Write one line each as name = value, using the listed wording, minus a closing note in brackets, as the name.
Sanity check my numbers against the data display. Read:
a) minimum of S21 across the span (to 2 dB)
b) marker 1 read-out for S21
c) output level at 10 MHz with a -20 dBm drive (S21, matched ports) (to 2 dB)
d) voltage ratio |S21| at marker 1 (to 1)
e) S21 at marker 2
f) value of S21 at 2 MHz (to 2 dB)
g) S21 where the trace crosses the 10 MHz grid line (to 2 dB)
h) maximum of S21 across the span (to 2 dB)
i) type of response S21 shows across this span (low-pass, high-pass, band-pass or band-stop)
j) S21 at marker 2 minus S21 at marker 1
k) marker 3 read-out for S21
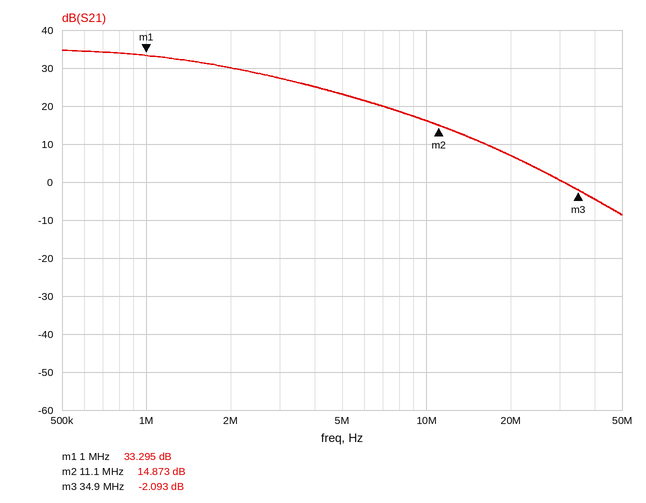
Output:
minimum of S21 across the span = -8 dB
marker 1 read-out for S21 = 33.295 dB
output level at 10 MHz with a -20 dBm drive (S21, matched ports) = -4 dBm
voltage ratio |S21| at marker 1 = 46
S21 at marker 2 = 14.873 dB
value of S21 at 2 MHz = 30 dB
S21 where the trace crosses the 10 MHz grid line = 16 dB
maximum of S21 across the span = 34 dB
type of response S21 shows across this span = low-pass
S21 at marker 2 minus S21 at marker 1 = -18.422 dB
marker 3 read-out for S21 = -2.093 dB
